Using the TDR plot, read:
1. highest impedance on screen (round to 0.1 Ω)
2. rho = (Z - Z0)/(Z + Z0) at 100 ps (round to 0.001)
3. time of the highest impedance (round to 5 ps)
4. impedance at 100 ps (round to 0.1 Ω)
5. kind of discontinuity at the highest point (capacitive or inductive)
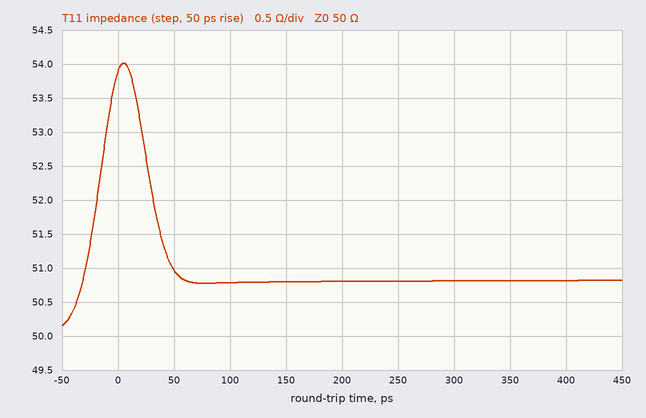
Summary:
54.0 Ω
+0.008
5 ps
50.8 Ω
inductive
